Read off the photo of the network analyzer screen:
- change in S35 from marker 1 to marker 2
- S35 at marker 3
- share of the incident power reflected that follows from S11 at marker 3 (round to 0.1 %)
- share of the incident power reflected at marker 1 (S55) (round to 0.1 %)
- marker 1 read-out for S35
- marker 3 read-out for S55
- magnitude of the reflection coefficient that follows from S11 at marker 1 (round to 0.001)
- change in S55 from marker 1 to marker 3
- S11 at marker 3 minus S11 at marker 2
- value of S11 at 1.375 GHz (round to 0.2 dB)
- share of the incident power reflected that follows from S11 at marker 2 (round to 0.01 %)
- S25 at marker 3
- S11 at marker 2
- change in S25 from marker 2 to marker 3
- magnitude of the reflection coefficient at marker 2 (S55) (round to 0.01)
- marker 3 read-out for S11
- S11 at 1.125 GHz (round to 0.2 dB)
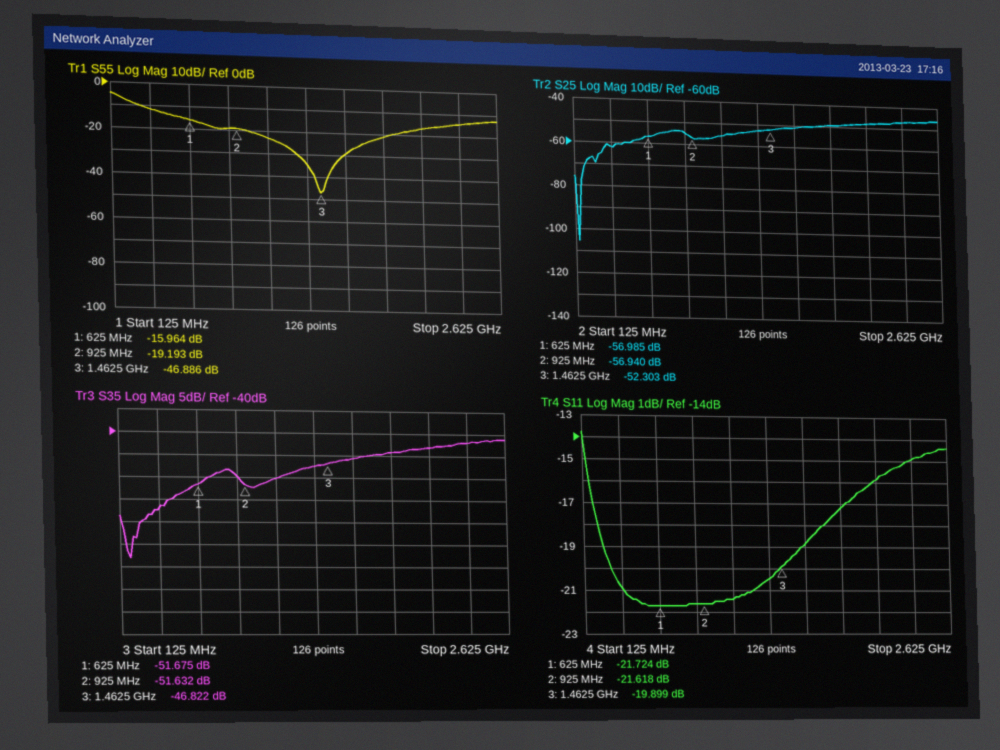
0.043 dB
-46.822 dB
1.0 %
2.5 %
-51.675 dB
-46.886 dB
0.082
-30.922 dB
1.719 dB
-20.4 dB
0.69 %
-52.303 dB
-21.618 dB
4.637 dB
0.11
-19.899 dB
-21.4 dB
